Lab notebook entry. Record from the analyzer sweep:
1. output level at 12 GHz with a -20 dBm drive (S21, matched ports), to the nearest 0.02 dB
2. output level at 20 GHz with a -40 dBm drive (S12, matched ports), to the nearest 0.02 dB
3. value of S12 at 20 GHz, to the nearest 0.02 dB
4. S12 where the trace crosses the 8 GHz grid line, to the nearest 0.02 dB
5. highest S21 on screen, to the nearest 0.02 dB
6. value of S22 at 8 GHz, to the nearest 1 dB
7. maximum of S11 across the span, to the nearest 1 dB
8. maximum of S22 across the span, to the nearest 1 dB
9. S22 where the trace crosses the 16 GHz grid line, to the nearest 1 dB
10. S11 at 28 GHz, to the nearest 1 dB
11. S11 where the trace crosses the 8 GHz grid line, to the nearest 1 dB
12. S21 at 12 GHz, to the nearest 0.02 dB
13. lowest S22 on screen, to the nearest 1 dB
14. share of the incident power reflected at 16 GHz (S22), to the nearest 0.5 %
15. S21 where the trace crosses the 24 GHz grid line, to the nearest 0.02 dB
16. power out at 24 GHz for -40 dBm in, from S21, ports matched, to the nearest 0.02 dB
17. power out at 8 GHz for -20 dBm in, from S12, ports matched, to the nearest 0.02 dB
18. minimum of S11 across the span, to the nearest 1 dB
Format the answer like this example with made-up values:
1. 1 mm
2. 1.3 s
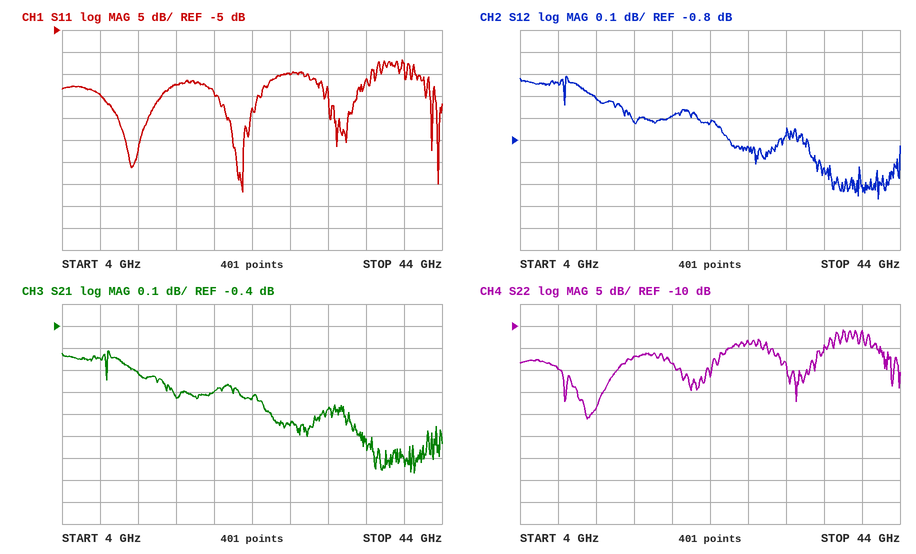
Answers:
1. -20.62 dBm
2. -40.70 dBm
3. -0.70 dB
4. -0.54 dB
5. -0.52 dB
6. -20 dB
7. -12 dB
8. -11 dB
9. -17 dB
10. -15 dB
11. -20 dB
12. -0.62 dB
13. -31 dB
14. 2.0 %
15. -0.72 dB
16. -40.72 dBm
17. -20.54 dBm
18. -42 dB
